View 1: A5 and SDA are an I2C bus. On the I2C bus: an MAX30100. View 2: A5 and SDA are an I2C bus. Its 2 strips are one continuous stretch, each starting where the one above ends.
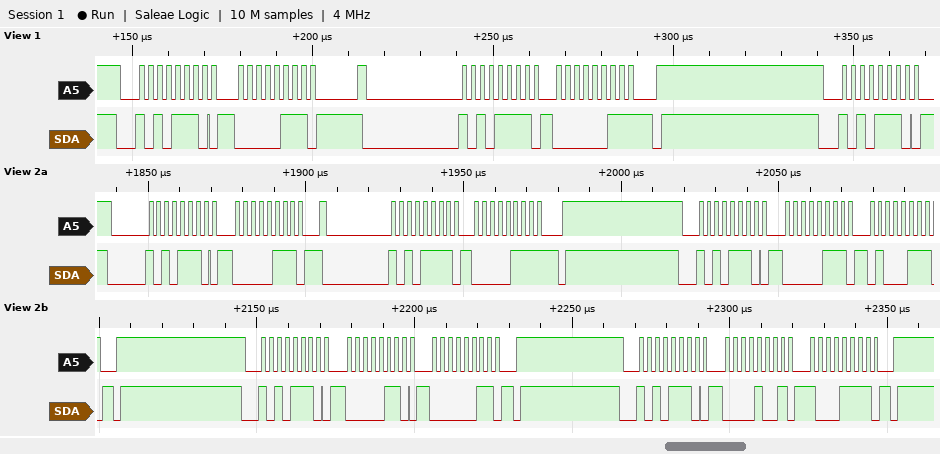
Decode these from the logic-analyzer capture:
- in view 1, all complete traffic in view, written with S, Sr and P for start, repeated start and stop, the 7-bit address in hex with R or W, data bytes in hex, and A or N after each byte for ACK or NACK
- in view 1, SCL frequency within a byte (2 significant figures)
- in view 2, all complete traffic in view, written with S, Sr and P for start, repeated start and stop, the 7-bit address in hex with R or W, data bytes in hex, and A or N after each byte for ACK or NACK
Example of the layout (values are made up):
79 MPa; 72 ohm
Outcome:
S 57W A 07 A Sr 57R A 03 N P S 57W A; 400 kHz; S 57W A 07 A Sr 57R A 07 N P S 57W A 07 A 47 A P S 57W A 06 A 03 A P S 57W A 09 A 8F A P
